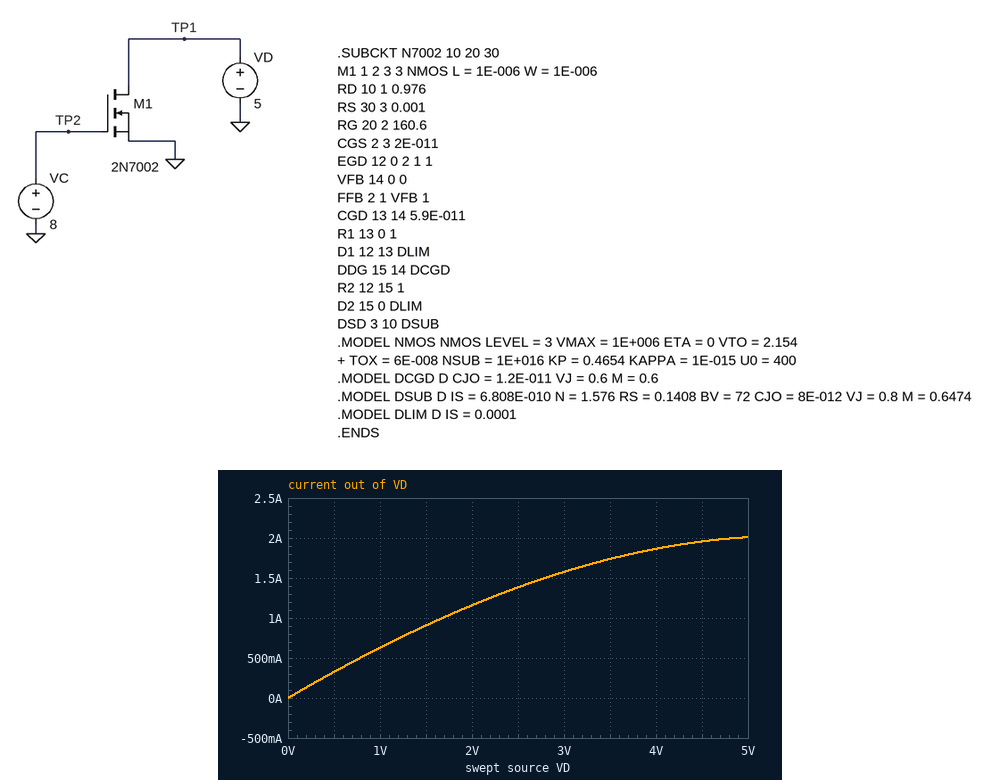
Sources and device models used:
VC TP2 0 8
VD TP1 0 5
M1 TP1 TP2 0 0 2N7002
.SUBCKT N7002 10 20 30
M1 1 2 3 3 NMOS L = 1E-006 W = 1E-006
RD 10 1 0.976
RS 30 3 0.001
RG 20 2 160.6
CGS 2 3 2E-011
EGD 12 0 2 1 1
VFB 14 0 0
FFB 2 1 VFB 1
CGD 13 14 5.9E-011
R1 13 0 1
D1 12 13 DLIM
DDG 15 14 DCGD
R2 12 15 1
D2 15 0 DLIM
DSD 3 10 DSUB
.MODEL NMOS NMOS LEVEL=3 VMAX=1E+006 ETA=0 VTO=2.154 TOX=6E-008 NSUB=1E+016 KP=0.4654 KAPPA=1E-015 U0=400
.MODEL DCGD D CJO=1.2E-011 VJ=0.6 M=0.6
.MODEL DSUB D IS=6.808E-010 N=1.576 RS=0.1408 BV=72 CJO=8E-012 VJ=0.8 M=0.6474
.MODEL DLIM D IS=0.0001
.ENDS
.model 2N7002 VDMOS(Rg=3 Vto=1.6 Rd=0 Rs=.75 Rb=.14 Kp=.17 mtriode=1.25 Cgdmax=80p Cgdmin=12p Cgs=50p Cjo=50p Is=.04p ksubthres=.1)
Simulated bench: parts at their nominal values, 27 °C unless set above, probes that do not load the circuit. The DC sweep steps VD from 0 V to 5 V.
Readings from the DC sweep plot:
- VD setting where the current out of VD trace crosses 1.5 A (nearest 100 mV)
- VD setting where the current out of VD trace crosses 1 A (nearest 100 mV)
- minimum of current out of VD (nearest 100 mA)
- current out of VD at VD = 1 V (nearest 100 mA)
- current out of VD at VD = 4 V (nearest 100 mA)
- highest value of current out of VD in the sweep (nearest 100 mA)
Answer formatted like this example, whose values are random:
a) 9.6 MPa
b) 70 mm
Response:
a) 2.8 V
b) 1.7 V
c) 0 A
d) 600 mA
e) 1.9 A
f) 2.0 A
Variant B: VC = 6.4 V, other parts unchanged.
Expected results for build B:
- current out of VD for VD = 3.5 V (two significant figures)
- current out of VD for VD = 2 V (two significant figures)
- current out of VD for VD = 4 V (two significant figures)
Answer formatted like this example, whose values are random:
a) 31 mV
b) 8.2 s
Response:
a) 1.2 A
b) 920 mA
c) 1.3 A
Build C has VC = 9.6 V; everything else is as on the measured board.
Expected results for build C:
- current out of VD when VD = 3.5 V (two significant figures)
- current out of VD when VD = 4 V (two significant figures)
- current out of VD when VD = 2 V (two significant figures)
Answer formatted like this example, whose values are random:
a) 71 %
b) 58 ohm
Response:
a) 2.1 A
b) 2.3 A
c) 1.3 A
